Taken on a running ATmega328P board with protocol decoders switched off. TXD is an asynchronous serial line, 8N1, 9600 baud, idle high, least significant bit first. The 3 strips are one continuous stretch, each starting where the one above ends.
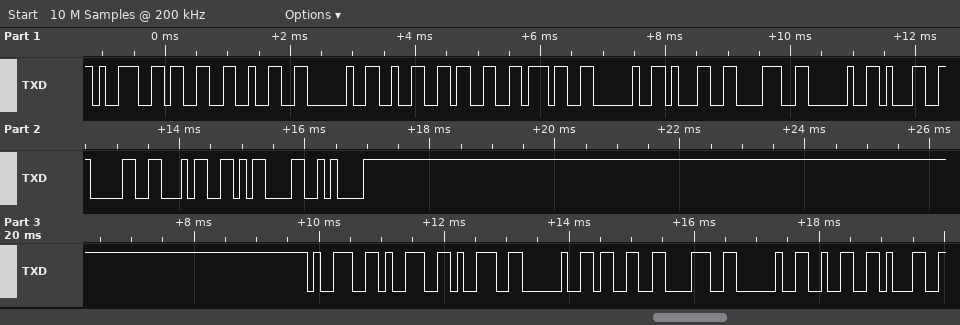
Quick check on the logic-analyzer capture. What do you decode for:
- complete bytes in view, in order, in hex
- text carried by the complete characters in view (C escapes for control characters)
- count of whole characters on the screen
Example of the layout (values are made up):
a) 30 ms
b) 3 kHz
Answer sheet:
a) 39 33 32 20 32 33 37 20 31 38 20 31 30 34 0D 0A 39 39 39 20 33 38 20 32 31
b) "932 237 18 104\r\n999 38 21"
c) 25
